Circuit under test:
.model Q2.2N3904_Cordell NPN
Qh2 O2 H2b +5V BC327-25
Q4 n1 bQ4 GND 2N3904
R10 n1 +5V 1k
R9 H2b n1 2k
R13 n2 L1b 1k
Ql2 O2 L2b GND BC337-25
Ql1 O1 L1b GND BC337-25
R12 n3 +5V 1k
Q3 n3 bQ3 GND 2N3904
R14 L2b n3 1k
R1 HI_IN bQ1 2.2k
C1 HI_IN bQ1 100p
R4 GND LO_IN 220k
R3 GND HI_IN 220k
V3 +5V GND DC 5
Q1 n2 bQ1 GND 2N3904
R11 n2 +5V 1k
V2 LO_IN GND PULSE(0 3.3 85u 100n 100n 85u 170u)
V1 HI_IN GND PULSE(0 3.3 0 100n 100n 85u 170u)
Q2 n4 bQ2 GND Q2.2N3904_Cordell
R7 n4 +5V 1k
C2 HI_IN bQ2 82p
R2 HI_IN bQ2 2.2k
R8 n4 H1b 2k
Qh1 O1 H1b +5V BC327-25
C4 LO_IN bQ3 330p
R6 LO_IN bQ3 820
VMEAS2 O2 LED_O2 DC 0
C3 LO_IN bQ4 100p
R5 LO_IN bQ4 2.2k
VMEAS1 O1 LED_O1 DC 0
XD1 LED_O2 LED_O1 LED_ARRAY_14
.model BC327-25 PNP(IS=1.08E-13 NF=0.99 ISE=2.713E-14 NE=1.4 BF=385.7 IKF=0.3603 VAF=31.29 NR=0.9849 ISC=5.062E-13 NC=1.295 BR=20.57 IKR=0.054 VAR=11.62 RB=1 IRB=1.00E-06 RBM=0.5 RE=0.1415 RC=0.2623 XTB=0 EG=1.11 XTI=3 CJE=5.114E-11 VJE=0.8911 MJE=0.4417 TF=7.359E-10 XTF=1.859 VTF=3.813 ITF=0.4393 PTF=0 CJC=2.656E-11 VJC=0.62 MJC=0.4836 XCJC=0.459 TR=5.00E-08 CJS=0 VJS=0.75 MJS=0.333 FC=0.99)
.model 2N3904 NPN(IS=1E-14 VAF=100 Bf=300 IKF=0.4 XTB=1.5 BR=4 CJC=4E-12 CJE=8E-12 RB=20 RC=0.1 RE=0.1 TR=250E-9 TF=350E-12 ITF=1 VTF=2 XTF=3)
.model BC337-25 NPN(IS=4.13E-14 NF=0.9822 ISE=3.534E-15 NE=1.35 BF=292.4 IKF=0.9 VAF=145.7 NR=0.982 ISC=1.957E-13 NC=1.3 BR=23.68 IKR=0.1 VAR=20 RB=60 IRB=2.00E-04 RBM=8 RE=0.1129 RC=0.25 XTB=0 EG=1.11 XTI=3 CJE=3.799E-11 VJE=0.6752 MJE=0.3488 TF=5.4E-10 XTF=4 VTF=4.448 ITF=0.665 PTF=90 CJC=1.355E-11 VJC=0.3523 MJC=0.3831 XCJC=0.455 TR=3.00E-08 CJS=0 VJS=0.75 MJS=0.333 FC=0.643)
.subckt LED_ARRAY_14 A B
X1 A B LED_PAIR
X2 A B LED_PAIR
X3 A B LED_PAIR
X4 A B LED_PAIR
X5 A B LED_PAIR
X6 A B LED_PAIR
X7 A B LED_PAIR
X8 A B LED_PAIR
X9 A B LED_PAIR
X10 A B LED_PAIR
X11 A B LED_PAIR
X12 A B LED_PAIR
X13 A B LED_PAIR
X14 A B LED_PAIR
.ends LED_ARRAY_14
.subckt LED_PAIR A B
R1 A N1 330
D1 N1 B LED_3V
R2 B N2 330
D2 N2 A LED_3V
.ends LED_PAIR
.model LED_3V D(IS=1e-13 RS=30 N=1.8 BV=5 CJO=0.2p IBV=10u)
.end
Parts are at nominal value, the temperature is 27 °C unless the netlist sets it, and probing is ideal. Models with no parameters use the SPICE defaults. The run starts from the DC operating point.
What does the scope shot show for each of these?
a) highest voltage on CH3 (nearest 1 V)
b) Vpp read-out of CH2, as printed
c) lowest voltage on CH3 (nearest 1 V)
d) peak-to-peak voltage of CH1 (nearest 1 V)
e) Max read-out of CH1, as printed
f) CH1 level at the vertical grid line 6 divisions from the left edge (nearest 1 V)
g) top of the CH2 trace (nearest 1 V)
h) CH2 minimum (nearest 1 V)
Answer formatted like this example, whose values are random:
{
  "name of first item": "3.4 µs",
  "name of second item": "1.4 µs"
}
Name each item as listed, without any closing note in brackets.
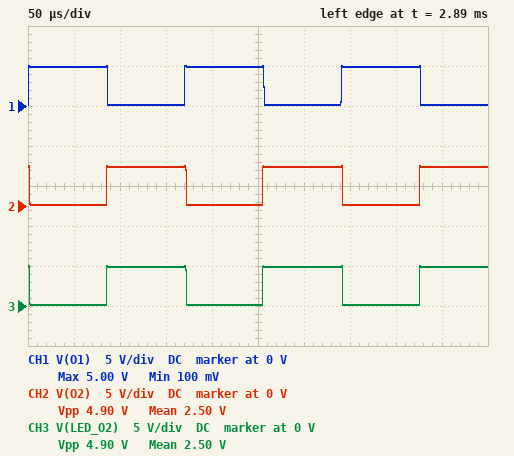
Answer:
{
  "highest voltage on CH3": "5 V",
  "Vpp read-out of CH2, as printed": "4.90 V",
  "lowest voltage on CH3": "0 V",
  "peak-to-peak voltage of CH1": "5 V",
  "Max read-out of CH1, as printed": "5.00 V",
  "CH1 level at the vertical grid line 6 divisions from the left edge": "0 V",
  "top of the CH2 trace": "5 V",
  "CH2 minimum": "0 V"
}
